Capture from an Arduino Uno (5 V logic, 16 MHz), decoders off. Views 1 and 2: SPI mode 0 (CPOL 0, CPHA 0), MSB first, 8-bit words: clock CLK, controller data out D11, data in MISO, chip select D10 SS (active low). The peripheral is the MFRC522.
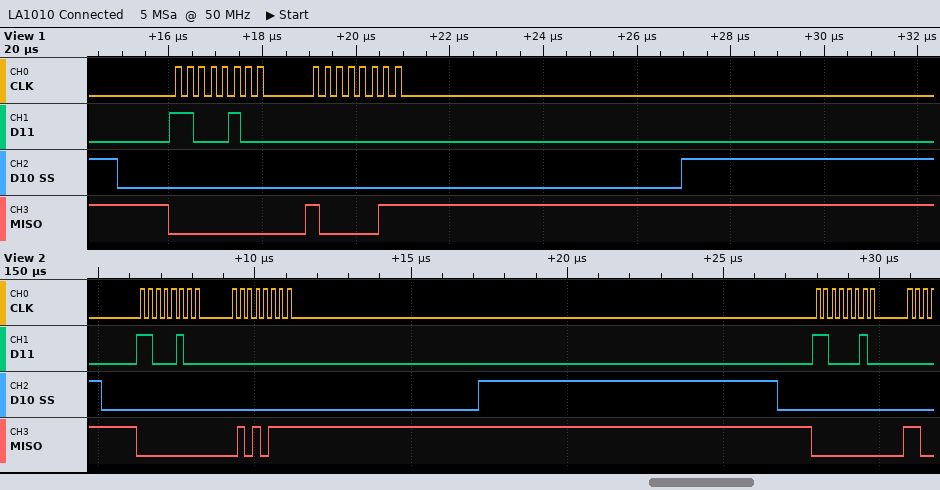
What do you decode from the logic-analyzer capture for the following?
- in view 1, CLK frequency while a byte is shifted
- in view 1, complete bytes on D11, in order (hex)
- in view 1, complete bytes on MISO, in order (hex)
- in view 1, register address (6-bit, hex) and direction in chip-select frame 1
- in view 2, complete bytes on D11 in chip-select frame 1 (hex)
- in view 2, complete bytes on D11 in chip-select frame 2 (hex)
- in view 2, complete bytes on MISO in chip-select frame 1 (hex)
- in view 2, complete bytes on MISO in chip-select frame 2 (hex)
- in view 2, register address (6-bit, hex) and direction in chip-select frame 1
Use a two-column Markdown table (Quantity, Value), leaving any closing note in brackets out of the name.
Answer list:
| Quantity | Value |
|---|---|
| in view 1, CLK frequency while a byte is shifted | 4 MHz |
| in view 1, complete bytes on D11, in order | 0xC4 0x00 |
| in view 1, complete bytes on MISO, in order | 0x00 0x83 |
| in view 1, register address (6-bit, hex) and direction in chip-select frame 1 | 0x22 read |
| in view 2, complete bytes on D11 in chip-select frame 1 | C4 00 |
| in view 2, complete bytes on D11 in chip-select frame 2 | C2 |
| in view 2, complete bytes on MISO in chip-select frame 1 | 00 57 |
| in view 2, complete bytes on MISO in chip-select frame 2 | 00 |
| in view 2, register address (6-bit, hex) and direction in chip-select frame 1 | 0x22 read |
